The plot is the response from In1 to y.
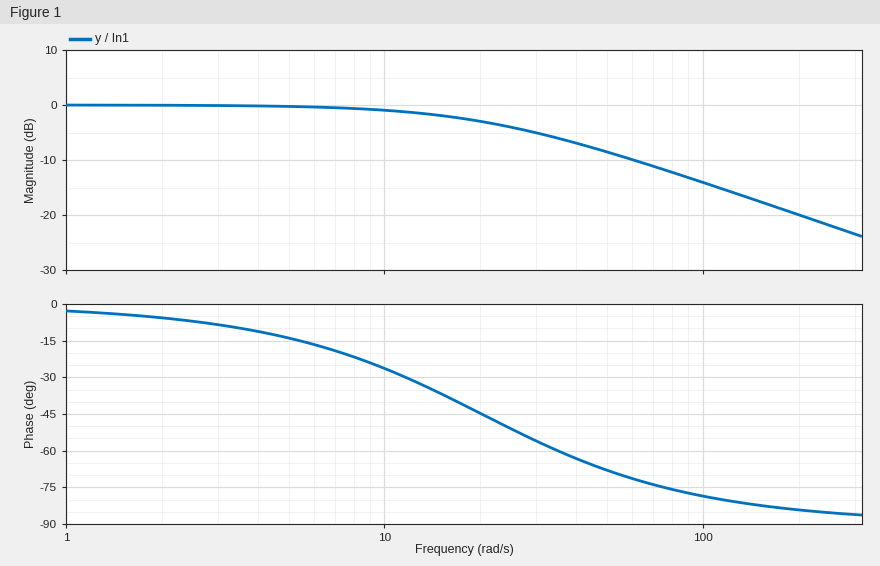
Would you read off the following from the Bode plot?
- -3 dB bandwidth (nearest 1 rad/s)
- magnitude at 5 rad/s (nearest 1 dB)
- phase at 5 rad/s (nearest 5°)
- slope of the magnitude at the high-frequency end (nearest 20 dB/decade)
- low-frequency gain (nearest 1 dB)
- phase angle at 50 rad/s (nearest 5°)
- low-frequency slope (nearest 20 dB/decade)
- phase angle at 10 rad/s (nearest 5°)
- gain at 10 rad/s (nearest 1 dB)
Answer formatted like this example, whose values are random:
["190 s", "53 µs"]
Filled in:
["20 rad/s", "0 dB", "-15°", "-20 dB/decade", "0 dB", "-70°", "0 dB/decade", "-25°", "-1 dB"]
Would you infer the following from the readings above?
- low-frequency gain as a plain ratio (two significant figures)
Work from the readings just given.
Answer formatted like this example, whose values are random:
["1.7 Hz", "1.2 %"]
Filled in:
["1.0"]
